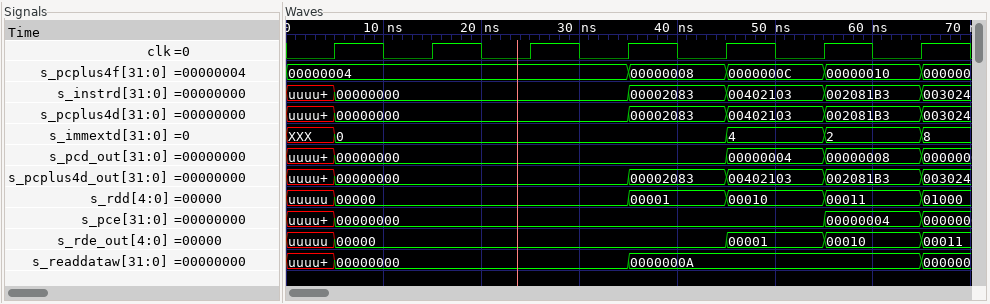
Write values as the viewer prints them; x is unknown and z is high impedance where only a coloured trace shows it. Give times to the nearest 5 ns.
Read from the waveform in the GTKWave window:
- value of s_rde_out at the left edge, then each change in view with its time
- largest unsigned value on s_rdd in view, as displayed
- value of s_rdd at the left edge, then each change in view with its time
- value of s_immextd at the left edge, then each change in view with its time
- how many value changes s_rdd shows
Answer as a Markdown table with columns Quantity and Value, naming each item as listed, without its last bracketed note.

| Quantity | Value |
|---|---|
| value of s_rde_out at the left edge, then each change in view with its time | uuuuu, 00000 at 5 ns, 00001 at 45 ns, 00010 at 55 ns, 00011 at 65 ns |
| largest unsigned value on s_rdd in view, as displayed | 01000 |
| value of s_rdd at the left edge, then each change in view with its time | uuuuu, 00000 at 5 ns, 00001 at 35 ns, 00010 at 45 ns, 00011 at 55 ns, 01000 at 65 ns |
| value of s_immextd at the left edge, then each change in view with its time | XXX, 0 at 5 ns, 4 at 45 ns, 2 at 55 ns, 8 at 65 ns |
| how many value changes s_rdd shows | 5 |
